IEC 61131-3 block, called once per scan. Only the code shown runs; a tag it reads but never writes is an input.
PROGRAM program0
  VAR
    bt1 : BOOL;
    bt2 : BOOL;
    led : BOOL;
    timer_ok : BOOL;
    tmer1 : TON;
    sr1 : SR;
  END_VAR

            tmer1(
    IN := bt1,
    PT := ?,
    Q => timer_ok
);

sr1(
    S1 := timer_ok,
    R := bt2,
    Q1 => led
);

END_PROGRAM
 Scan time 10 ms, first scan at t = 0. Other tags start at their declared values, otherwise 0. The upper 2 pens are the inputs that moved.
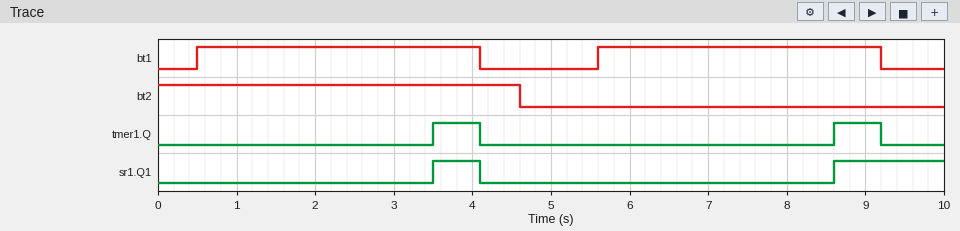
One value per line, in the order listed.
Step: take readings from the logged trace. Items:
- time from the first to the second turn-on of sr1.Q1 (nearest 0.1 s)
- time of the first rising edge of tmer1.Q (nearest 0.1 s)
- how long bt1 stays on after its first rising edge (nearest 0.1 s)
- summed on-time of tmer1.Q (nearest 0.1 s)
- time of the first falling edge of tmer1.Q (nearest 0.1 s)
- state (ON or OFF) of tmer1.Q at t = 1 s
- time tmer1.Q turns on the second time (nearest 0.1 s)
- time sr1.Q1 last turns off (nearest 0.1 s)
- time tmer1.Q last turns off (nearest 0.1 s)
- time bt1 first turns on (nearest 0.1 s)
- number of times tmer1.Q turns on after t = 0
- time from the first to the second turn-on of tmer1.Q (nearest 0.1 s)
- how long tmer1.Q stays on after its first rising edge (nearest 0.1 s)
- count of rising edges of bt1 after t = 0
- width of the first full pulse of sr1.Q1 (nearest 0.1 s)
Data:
5.1 s
3.5 s
3.6 s
1.2 s
4.1 s
OFF
8.6 s
4.1 s
9.2 s
0.5 s
2
5.1 s
0.6 s
2
0.6 s
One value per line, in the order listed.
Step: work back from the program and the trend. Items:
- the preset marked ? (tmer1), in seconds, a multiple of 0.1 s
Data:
3.0 s
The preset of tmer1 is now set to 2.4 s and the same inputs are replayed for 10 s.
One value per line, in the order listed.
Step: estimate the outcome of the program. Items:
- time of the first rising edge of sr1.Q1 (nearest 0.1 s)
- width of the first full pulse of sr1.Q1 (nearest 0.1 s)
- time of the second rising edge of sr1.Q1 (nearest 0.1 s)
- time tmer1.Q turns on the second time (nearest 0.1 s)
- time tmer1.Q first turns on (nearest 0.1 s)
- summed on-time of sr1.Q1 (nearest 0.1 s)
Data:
2.9 s
1.2 s
8.0 s
8.0 s
2.9 s
3.2 s
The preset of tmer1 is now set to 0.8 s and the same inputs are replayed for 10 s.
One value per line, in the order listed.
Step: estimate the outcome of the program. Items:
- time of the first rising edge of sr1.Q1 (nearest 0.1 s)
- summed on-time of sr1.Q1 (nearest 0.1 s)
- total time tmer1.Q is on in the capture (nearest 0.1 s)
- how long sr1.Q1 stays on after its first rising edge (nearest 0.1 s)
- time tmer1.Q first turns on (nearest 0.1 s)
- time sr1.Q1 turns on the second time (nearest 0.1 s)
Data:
1.3 s
6.4 s
5.6 s
2.8 s
1.3 s
6.4 s
